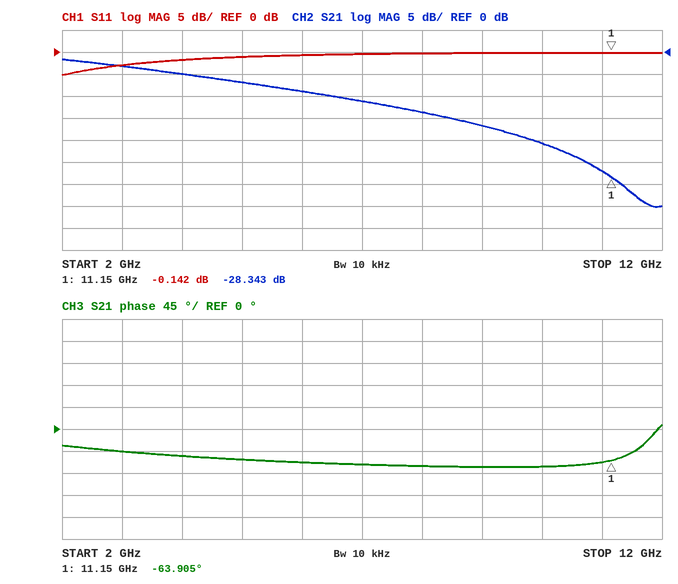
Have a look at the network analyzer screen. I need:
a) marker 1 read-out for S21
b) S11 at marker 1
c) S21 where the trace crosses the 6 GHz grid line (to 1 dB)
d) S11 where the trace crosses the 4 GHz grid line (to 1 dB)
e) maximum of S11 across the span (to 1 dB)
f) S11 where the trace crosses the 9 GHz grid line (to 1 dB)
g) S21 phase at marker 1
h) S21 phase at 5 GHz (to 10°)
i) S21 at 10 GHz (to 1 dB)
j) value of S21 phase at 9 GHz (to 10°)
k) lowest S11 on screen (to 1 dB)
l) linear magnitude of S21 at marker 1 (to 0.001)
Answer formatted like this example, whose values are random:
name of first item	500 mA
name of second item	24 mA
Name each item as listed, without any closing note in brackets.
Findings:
marker 1 read-out for S21	-28.343 dB
S11 at marker 1	-0.142 dB
S21 where the trace crosses the 6 GHz grid line	-9 dB
S11 where the trace crosses the 4 GHz grid line	-2 dB
maximum of S11 across the span	0 dB
S11 where the trace crosses the 9 GHz grid line	0 dB
S21 phase at marker 1	-63.905°
S21 phase at 5 GHz	-60°
S21 at 10 GHz	-21 dB
value of S21 phase at 9 GHz	-80°
lowest S11 on screen	-5 dB
linear magnitude of S21 at marker 1	0.038
